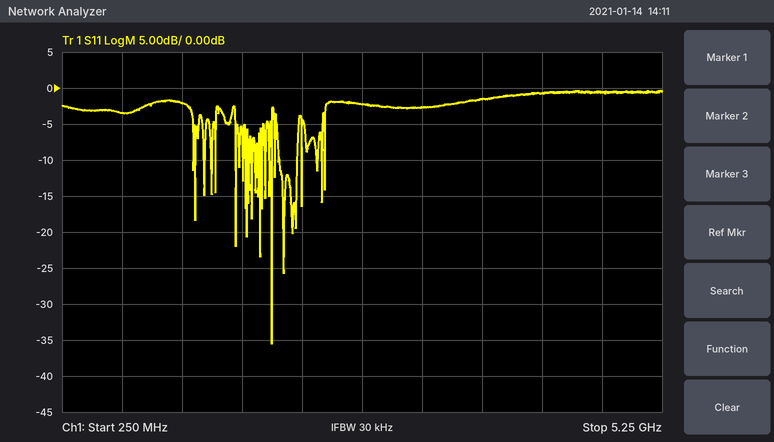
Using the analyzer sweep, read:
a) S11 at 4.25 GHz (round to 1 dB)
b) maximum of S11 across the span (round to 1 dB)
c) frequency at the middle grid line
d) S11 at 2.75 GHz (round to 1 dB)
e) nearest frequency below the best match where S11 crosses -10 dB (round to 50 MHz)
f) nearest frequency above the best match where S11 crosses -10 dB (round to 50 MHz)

-1 dB
0 dB
2.75 GHz
-2 dB
2.00 GHz
2.00 GHz
